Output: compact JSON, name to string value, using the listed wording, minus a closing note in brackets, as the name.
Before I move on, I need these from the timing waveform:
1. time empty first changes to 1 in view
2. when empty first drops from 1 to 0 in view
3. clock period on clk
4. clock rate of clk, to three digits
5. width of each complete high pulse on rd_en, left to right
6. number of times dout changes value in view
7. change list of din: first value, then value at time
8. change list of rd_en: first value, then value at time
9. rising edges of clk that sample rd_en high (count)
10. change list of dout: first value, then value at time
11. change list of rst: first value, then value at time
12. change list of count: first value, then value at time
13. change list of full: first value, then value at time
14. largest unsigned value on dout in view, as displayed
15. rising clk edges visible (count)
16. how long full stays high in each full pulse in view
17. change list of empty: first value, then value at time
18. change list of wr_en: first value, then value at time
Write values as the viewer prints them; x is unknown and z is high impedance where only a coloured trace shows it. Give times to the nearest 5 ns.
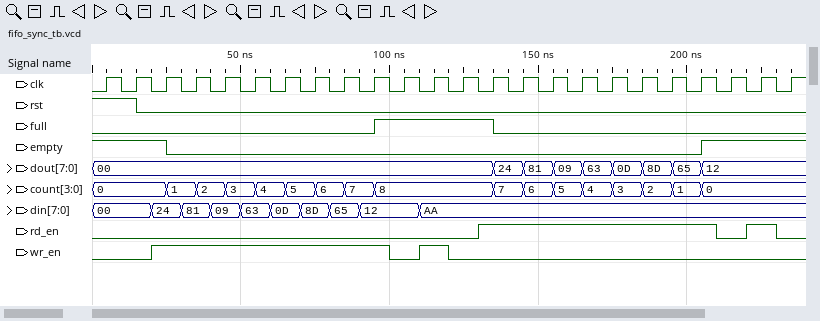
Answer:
{"time empty first changes to 1 in view": "205 ns", "when empty first drops from 1 to 0 in view": "25 ns", "clock period on clk": "10 ns", "clock rate of clk, to three digits": "100 MHz", "width of each complete high pulse on rd_en, left to right": "80 ns, 10 ns", "number of times dout changes value in view": "8", "change list of din: first value, then value at time": "00, 24 at 20 ns, 81 at 30 ns, 09 at 40 ns, 63 at 50 ns, 0D at 60 ns, 8D at 70 ns, 65 at 80 ns, 12 at 90 ns, AA at 110 ns", "change list of rd_en: first value, then value at time": "0, 1 at 130 ns, 0 at 210 ns, 1 at 220 ns, 0 at 230 ns", "rising edges of clk that sample rd_en high": "9", "change list of dout: first value, then value at time": "00, 24 at 135 ns, 81 at 145 ns, 09 at 155 ns, 63 at 165 ns, 0D at 175 ns, 8D at 185 ns, 65 at 195 ns, 12 at 205 ns", "change list of rst: first value, then value at time": "1, 0 at 15 ns", "change list of count: first value, then value at time": "0, 1 at 25 ns, 2 at 35 ns, 3 at 45 ns, 4 at 55 ns, 5 at 65 ns, 6 at 75 ns, 7 at 85 ns, 8 at 95 ns, 7 at 135 ns, 6 at 145 ns, 5 at 155 ns, 4 at 165 ns, 3 at 175 ns, 2 at 185 ns, 1 at 195 ns, 0 at 205 ns", "change list of full: first value, then value at time": "0, 1 at 95 ns, 0 at 135 ns", "largest unsigned value on dout in view, as displayed": "8D", "rising clk edges visible": "24", "how long full stays high in each full pulse in view": "40 ns", "change list of empty: first value, then value at time": "1, 0 at 25 ns, 1 at 205 ns", "change list of wr_en: first value, then value at time": "0, 1 at 20 ns, 0 at 100 ns, 1 at 110 ns, 0 at 120 ns"}
